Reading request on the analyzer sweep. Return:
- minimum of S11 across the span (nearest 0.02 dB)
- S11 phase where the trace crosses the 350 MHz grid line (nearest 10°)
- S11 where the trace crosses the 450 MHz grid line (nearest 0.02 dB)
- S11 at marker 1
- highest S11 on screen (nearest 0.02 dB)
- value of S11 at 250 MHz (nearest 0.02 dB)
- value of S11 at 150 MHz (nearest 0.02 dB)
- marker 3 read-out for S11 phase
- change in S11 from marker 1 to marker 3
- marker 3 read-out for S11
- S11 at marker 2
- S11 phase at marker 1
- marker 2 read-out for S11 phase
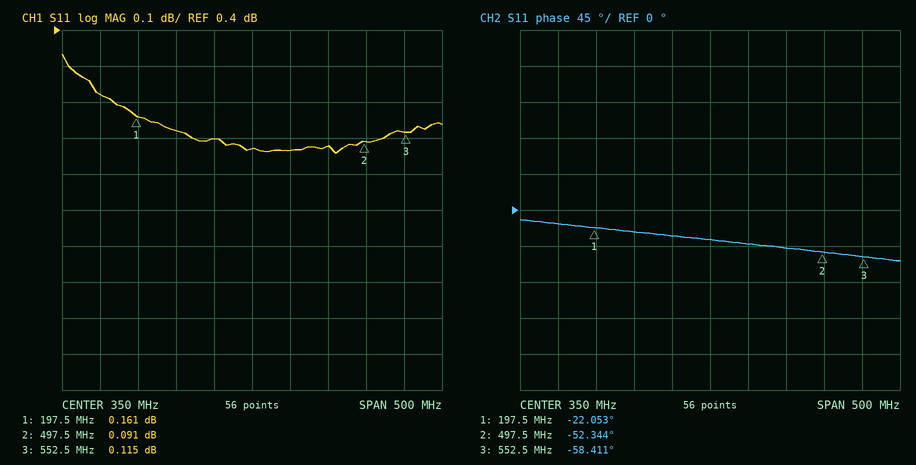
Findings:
0.06 dB
-40°
0.08 dB
0.161 dB
0.34 dB
0.12 dB
0.22 dB
-58.411°
-0.046 dB
0.115 dB
0.091 dB
-22.053°
-52.344°
